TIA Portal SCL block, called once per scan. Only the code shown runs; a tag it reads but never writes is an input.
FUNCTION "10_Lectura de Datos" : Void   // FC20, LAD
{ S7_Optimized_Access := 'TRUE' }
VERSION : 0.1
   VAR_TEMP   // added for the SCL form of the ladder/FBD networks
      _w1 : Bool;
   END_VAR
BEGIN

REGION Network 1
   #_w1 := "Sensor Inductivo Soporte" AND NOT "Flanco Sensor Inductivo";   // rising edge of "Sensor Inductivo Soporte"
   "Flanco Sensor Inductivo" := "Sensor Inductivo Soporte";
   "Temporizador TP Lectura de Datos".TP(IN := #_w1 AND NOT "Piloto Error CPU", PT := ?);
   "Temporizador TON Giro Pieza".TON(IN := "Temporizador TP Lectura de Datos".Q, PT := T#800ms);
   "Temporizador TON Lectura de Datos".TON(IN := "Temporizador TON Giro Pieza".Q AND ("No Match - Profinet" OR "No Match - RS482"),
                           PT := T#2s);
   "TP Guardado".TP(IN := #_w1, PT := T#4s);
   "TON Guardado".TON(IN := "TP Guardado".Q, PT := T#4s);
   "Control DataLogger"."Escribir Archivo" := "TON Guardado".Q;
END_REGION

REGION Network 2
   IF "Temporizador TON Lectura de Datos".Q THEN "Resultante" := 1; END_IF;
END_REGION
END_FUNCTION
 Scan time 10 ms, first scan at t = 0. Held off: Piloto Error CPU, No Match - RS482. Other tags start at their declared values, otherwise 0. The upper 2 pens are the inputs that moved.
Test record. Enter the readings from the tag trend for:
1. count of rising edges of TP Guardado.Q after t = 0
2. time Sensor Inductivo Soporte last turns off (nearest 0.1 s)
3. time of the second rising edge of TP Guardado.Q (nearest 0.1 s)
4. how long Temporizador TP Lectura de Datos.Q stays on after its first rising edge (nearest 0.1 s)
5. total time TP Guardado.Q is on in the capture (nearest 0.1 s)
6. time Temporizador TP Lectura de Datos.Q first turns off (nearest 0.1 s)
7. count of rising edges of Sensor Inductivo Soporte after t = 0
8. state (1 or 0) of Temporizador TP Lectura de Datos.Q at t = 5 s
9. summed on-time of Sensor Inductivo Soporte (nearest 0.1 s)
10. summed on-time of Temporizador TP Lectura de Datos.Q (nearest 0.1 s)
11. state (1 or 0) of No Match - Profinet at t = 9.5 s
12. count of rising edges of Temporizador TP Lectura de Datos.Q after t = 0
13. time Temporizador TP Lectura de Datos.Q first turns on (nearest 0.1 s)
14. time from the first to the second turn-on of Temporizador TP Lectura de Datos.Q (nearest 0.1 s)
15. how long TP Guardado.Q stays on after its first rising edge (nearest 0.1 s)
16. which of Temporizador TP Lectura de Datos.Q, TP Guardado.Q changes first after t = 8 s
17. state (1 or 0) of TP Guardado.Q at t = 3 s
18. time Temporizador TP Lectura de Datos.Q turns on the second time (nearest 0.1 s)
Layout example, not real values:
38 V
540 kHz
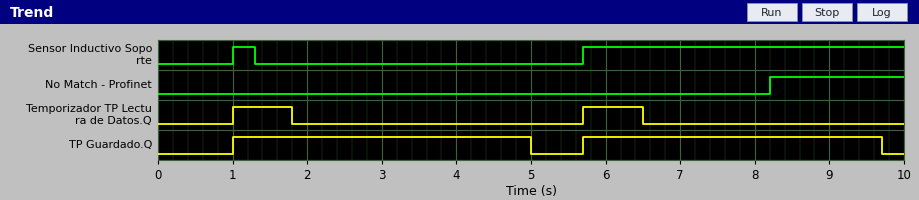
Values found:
2
1.3 s
5.7 s
0.8 s
8.0 s
1.8 s
2
0
4.6 s
1.6 s
1
2
1.0 s
4.7 s
4.0 s
TP Guardado.Q
1
5.7 s
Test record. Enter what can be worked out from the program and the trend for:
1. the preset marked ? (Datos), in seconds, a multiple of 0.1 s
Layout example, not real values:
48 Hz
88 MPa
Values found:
0.8 s
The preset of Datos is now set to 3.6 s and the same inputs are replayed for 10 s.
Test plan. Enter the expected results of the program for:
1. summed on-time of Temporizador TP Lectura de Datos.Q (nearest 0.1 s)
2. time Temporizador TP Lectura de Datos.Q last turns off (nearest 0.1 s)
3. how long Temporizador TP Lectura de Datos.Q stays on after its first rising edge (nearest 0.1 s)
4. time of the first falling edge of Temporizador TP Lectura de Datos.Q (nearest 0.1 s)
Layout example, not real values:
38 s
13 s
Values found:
7.2 s
9.3 s
3.6 s
4.6 s
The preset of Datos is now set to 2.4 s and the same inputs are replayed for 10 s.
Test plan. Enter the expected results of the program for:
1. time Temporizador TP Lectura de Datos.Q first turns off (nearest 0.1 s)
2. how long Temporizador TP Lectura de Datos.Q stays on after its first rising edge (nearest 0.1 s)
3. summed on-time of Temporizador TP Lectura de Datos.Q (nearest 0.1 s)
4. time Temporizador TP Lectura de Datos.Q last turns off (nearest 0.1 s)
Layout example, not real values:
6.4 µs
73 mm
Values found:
3.4 s
2.4 s
4.8 s
8.1 s
